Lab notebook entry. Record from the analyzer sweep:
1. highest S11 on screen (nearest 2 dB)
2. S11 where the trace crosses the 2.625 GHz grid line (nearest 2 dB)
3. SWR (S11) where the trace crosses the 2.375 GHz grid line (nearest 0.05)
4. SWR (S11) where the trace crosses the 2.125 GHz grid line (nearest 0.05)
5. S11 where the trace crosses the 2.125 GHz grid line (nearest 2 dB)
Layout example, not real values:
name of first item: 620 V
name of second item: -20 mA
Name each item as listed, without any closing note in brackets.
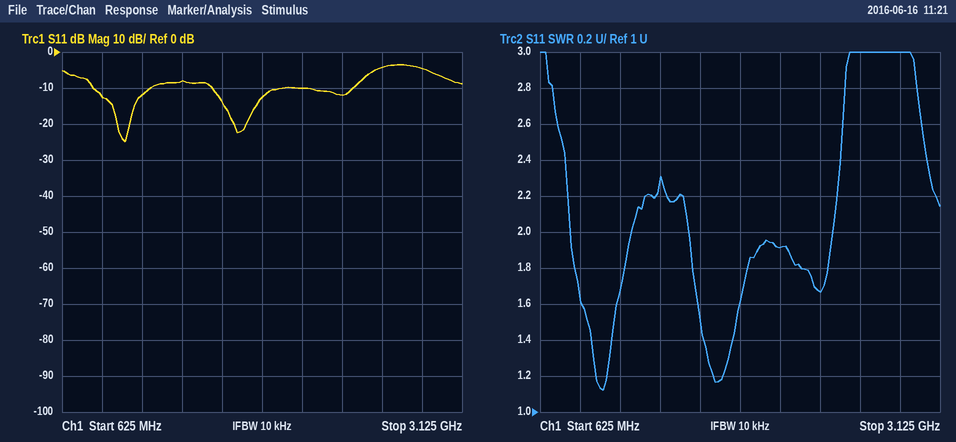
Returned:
highest S11 on screen: -4 dB
S11 where the trace crosses the 2.625 GHz grid line: -4 dB
SWR (S11) where the trace crosses the 2.375 GHz grid line: 1.65
SWR (S11) where the trace crosses the 2.125 GHz grid line: 1.90
S11 where the trace crosses the 2.125 GHz grid line: -10 dB
